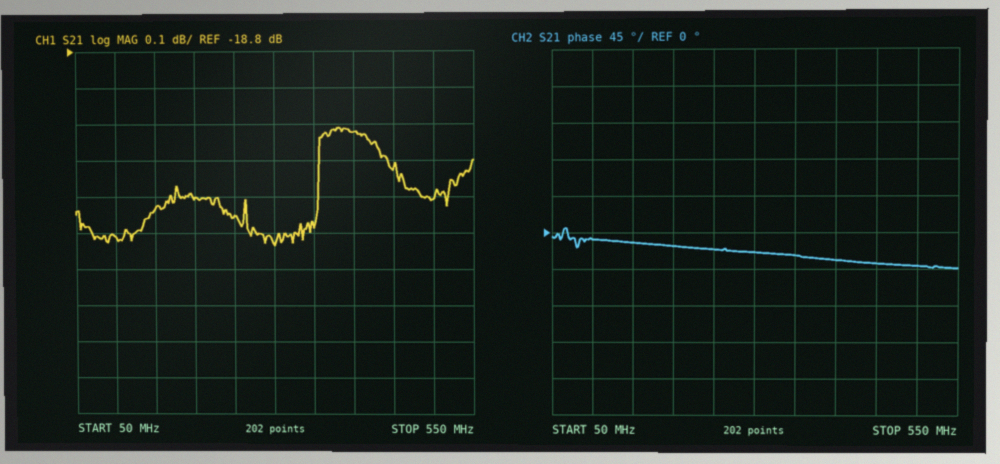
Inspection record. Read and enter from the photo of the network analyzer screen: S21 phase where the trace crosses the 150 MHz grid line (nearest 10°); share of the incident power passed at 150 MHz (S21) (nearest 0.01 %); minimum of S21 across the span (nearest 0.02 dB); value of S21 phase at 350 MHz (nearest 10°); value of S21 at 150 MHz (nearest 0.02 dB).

-10°
1.19 %
-19.34 dB
-30°
-19.24 dB
